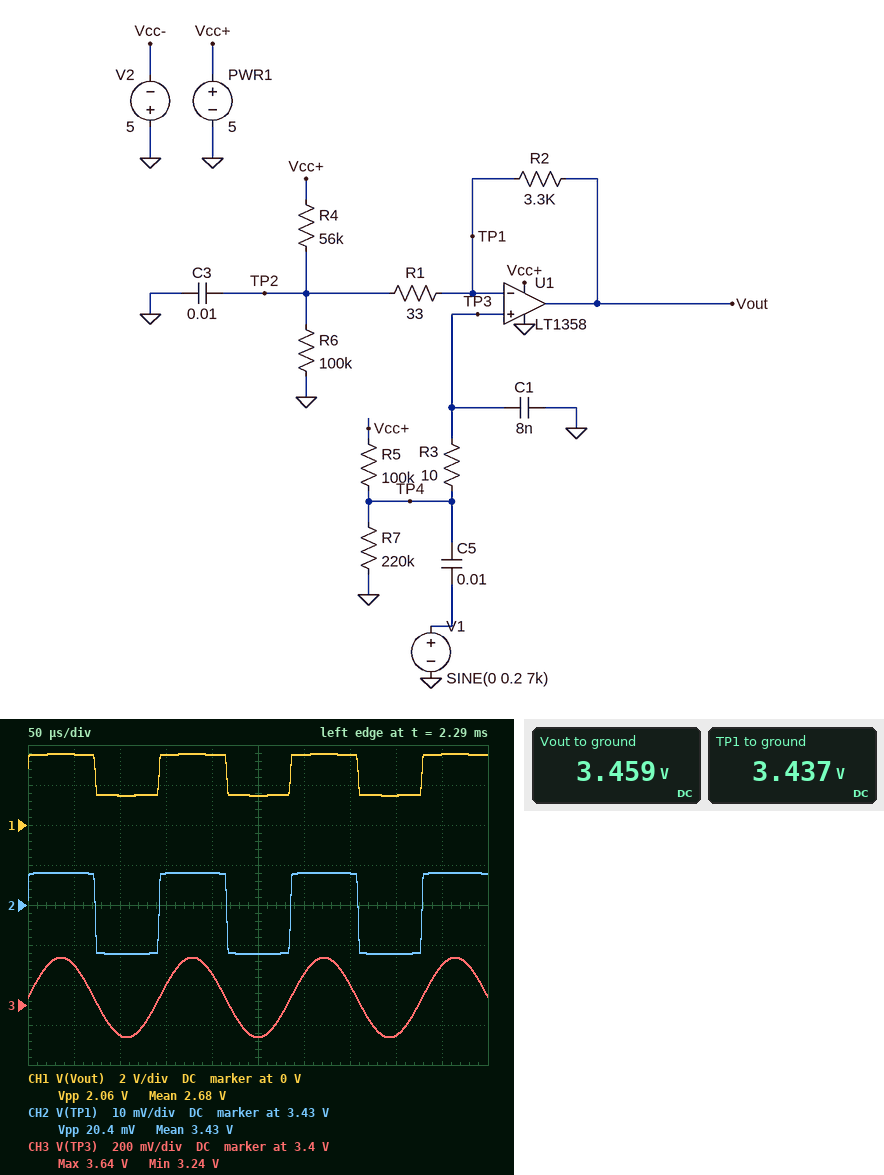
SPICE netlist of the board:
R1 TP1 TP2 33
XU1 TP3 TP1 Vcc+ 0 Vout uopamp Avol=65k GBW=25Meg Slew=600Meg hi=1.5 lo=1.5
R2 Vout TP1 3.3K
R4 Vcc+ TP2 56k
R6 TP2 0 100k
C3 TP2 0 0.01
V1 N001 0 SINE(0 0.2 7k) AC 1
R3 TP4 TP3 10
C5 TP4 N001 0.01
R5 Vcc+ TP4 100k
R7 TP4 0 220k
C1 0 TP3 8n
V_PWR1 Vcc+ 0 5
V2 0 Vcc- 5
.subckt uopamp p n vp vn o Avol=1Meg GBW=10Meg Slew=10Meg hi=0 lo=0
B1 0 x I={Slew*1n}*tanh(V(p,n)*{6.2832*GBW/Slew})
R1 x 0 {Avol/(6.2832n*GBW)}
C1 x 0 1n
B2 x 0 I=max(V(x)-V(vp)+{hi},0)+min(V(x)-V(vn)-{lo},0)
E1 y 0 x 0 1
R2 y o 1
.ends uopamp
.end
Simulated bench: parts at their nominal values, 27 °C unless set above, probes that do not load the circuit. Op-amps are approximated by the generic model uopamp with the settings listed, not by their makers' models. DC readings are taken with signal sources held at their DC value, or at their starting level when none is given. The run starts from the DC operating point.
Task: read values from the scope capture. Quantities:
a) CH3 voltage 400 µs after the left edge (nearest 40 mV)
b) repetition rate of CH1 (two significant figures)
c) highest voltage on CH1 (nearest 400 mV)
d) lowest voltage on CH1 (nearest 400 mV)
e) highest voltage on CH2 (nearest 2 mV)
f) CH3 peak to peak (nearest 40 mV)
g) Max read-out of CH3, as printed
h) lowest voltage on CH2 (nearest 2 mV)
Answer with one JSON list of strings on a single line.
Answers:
["3.24 V", "7.0 kHz", "3.6 V", "1.6 V", "3.438 V", "400 mV", "3.64 V", "3.418 V"]
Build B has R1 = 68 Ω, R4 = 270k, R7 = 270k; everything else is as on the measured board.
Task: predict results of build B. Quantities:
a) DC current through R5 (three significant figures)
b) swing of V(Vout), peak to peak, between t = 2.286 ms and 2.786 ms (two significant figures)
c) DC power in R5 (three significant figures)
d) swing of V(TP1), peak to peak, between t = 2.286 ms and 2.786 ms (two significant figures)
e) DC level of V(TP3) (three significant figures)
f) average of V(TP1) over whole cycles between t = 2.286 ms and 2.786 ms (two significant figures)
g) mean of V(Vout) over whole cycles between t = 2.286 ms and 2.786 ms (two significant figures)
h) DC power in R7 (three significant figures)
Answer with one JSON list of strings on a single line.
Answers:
["13.5 µA", "62 mV", "18.3 µW", "1.3 mV", "3.65 V", "3.4 V", "3.5 V", "49.3 µW"]
